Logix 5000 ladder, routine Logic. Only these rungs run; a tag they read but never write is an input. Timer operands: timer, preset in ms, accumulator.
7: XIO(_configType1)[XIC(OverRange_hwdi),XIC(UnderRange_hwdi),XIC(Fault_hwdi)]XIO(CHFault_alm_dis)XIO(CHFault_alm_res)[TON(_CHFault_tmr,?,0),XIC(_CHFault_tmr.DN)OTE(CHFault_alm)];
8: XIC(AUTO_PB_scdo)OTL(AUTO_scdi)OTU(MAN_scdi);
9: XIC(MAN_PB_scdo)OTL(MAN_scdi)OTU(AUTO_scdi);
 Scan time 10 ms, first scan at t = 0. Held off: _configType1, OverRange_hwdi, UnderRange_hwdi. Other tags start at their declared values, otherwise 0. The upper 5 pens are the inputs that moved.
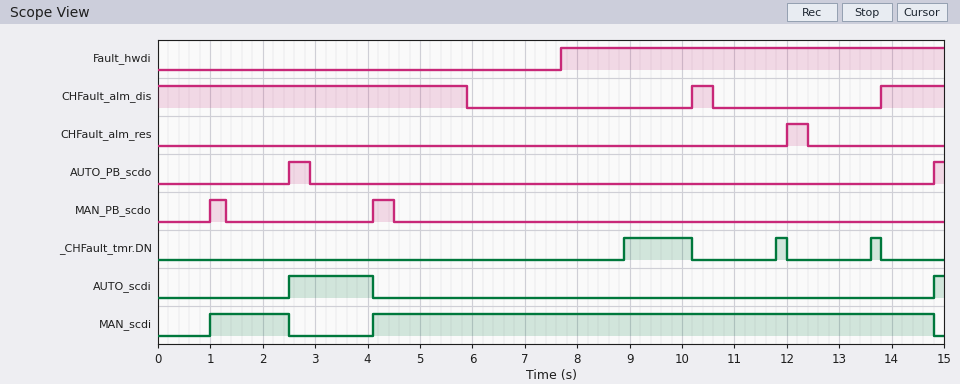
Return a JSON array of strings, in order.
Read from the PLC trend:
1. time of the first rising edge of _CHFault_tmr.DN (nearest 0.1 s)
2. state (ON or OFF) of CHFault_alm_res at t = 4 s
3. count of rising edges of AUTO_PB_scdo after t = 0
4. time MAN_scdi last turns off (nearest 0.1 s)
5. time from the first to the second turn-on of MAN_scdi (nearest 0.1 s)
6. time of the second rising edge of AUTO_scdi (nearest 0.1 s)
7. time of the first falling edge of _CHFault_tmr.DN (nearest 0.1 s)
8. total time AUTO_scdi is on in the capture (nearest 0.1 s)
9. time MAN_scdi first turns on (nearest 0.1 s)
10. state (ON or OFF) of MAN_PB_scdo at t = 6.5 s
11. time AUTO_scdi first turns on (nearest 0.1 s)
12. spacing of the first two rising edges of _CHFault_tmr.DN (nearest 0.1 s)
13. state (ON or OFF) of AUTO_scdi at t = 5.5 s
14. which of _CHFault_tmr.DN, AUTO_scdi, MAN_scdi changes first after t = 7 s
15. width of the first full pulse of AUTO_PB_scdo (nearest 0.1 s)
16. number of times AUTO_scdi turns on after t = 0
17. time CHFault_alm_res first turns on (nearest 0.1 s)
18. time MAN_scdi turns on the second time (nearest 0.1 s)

["8.9 s", "OFF", "2", "14.8 s", "3.1 s", "14.8 s", "10.2 s", "1.8 s", "1.0 s", "OFF", "2.5 s", "2.9 s", "OFF", "_CHFault_tmr.DN", "0.4 s", "2", "12.0 s", "4.1 s"]
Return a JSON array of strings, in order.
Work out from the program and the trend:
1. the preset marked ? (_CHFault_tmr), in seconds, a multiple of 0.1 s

["1.2 s"]
